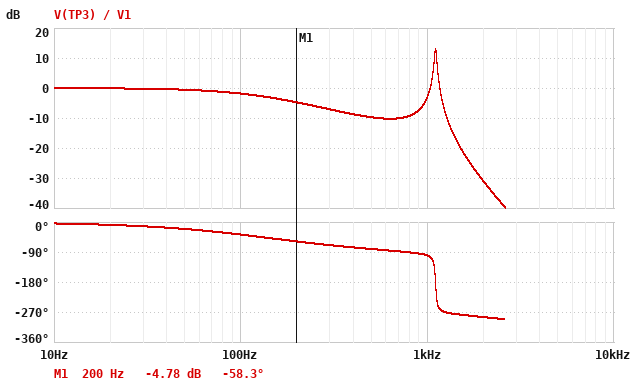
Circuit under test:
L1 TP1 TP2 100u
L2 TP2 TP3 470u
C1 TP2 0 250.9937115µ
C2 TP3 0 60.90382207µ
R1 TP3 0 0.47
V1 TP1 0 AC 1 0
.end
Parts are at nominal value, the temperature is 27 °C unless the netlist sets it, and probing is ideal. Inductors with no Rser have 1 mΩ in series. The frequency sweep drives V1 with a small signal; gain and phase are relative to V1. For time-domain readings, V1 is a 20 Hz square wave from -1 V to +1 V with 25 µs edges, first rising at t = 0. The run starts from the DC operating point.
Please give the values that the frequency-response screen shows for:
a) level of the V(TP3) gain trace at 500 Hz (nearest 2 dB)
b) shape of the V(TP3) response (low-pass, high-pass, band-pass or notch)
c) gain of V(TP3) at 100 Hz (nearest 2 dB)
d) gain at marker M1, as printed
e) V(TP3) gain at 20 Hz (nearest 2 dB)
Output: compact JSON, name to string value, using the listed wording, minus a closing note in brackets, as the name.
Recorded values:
{"level of the V(TP3) gain trace at 500 Hz": "-10 dB", "shape of the V(TP3) response": "band-pass", "gain of V(TP3) at 100 Hz": "-2 dB", "gain at marker M1, as printed": "-4.78 dB", "V(TP3) gain at 20 Hz": "0 dB"}
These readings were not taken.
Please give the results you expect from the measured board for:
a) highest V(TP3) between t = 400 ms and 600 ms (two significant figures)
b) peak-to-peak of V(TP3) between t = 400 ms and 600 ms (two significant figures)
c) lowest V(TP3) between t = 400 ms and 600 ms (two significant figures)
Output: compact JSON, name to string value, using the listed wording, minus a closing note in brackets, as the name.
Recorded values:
{"highest V(TP3) between t = 400 ms and 600 ms": "1.1 V", "peak-to-peak of V(TP3) between t = 400 ms and 600 ms": "2.2 V", "lowest V(TP3) between t = 400 ms and 600 ms": "-1.1 V"}
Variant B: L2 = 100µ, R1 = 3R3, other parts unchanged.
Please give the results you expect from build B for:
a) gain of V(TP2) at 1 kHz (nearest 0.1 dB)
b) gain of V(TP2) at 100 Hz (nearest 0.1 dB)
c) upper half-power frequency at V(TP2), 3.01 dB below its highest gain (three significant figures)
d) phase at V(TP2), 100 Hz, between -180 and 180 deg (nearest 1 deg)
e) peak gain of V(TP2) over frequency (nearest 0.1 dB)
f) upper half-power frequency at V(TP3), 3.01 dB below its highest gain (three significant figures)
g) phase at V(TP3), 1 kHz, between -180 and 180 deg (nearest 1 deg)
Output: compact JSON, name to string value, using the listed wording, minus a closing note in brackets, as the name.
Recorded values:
{"gain of V(TP2) at 1 kHz": "8.2 dB", "gain of V(TP2) at 100 Hz": "0.1 dB", "upper half-power frequency at V(TP2), 3.01 dB below its highest gain": "983 Hz", "phase at V(TP2), 100 Hz, between -180 and 180 deg": "-1 deg", "peak gain of V(TP2) over frequency": "12.0 dB", "upper half-power frequency at V(TP3), 3.01 dB below its highest gain": "993 Hz", "phase at V(TP3), 1 kHz, between -180 and 180 deg": "-140 deg"}
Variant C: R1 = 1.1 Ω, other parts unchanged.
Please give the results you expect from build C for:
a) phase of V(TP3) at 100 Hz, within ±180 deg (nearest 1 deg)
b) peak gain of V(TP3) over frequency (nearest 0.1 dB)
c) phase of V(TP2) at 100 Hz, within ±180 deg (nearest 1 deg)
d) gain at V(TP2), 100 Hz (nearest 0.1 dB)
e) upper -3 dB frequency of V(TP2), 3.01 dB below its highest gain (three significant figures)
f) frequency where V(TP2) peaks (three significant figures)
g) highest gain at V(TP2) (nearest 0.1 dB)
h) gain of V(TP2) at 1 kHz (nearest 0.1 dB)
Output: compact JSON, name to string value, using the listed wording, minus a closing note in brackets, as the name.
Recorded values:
{"phase of V(TP3) at 100 Hz, within ±180 deg": "-18 deg", "peak gain of V(TP3) over frequency": "13.3 dB", "phase of V(TP2) at 100 Hz, within ±180 deg": "-3 deg", "gain at V(TP2), 100 Hz": "0 dB", "upper -3 dB frequency of V(TP2), 3.01 dB below its highest gain": "1.14 kHz", "frequency where V(TP2) peaks": "1.11 kHz", "highest gain at V(TP2)": "22.9 dB", "gain of V(TP2) at 1 kHz": "12.4 dB"}
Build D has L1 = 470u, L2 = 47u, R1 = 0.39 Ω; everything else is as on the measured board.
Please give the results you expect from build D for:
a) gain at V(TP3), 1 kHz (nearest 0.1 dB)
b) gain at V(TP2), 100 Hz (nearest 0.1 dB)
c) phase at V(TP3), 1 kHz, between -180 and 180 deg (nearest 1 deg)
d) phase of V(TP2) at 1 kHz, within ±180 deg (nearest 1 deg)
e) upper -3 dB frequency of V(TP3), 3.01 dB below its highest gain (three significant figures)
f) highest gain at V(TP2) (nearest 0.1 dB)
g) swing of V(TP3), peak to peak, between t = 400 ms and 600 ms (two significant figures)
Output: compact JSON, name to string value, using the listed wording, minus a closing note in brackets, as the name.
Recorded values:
{"gain at V(TP3), 1 kHz": "-16.3 dB", "gain at V(TP2), 100 Hz": "-2.0 dB", "phase at V(TP3), 1 kHz, between -180 and 180 deg": "-132 deg", "phase of V(TP2) at 1 kHz, within ±180 deg": "-92 deg", "upper -3 dB frequency of V(TP3), 3.01 dB below its highest gain": "133 Hz", "highest gain at V(TP2)": "0 dB", "swing of V(TP3), peak to peak, between t = 400 ms and 600 ms": "2.0 V"}
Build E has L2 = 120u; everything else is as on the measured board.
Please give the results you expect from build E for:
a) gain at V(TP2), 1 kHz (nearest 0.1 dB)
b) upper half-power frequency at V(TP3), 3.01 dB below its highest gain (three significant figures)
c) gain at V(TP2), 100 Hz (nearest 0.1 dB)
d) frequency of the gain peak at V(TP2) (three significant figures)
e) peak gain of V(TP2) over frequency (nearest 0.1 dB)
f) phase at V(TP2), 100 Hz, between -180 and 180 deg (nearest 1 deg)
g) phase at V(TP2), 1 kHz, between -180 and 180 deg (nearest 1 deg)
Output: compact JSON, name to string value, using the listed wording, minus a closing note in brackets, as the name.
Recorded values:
{"gain at V(TP2), 1 kHz": "2.1 dB", "upper half-power frequency at V(TP3), 3.01 dB below its highest gain": "1.46 kHz", "gain at V(TP2), 100 Hz": "-0.2 dB", "frequency of the gain peak at V(TP2)": "1.34 kHz", "peak gain of V(TP2) over frequency": "8.6 dB", "phase at V(TP2), 100 Hz, between -180 and 180 deg": "-7 deg", "phase at V(TP2), 1 kHz, between -180 and 180 deg": "-34 deg"}
